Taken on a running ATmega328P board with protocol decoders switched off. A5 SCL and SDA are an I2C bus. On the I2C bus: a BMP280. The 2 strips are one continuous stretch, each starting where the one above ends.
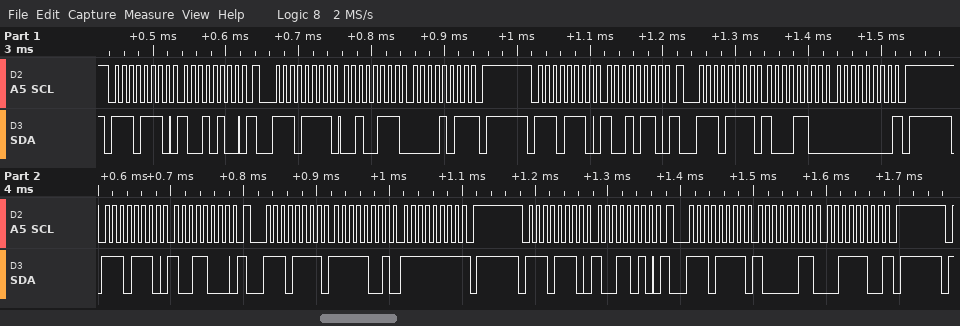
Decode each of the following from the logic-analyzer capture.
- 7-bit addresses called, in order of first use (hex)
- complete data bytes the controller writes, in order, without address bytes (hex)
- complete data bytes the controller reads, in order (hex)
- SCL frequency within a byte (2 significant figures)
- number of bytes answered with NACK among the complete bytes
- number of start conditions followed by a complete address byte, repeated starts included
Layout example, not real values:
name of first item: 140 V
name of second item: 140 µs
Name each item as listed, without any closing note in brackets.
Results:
7-bit addresses called, in order of first use: 0x77
complete data bytes the controller writes, in order, without address bytes: 94 96 98 9A
complete data bytes the controller reads, in order: 27 0B 8C 00 F9 FF 83 3C
SCL frequency within a byte: 100 kHz
number of bytes answered with NACK among the complete bytes: 4
number of start conditions followed by a complete address byte, repeated starts included: 8
